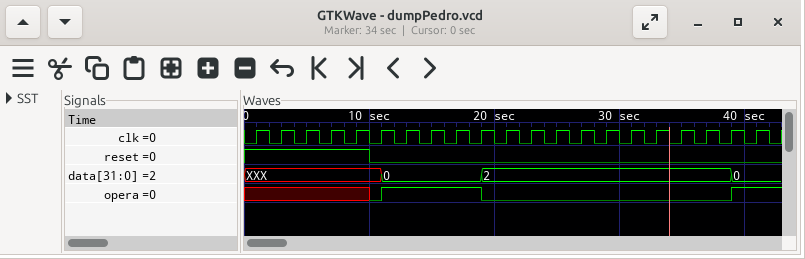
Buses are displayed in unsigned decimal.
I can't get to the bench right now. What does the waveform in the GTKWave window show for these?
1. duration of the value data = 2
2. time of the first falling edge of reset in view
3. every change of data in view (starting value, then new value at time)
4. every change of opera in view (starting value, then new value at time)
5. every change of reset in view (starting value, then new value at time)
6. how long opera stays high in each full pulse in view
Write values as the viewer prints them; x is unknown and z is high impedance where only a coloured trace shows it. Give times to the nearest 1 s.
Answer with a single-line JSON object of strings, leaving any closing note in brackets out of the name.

{"duration of the value data = 2": "20 s", "time of the first falling edge of reset in view": "10 s", "every change of data in view": "XXX, 0 at 11 s, 2 at 19 s, 0 at 39 s", "every change of opera in view": "x, 0 at 10 s, 1 at 11 s, 0 at 19 s, 1 at 39 s", "every change of reset in view": "1, 0 at 10 s", "how long opera stays high in each full pulse in view": "8 s"}
